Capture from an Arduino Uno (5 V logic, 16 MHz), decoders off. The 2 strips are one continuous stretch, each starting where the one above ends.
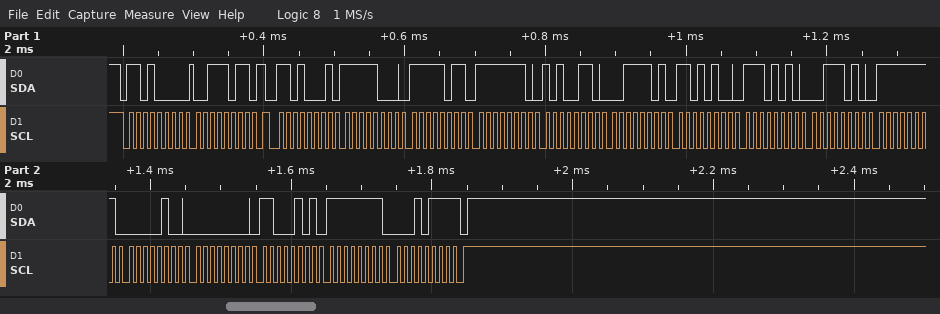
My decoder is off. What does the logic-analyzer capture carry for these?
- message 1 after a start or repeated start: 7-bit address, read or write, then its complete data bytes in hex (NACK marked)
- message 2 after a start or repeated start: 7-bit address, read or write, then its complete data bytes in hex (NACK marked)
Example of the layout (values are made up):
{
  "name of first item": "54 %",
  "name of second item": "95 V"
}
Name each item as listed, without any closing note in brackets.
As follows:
{
  "message 1 after a start or repeated start: 7-bit address, read or write, then its complete data bytes in hex": "0x68 write: 3B",
  "message 2 after a start or repeated start: 7-bit address, read or write, then its complete data bytes in hex": "0x68 read: F8 FB FE A6 3D D4 EA 3A FF 04 00 C5 FF 17 NACK"
}
